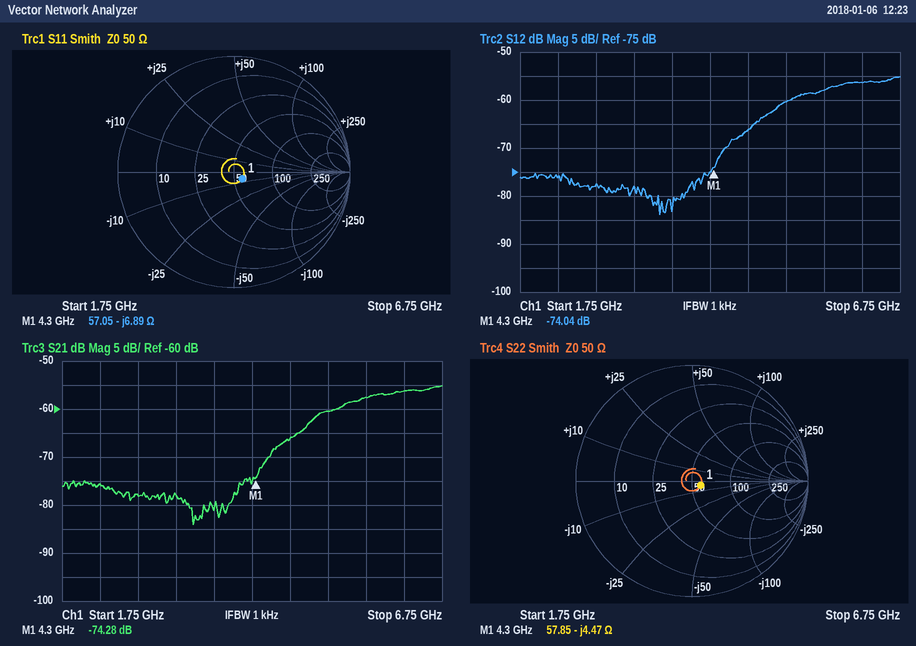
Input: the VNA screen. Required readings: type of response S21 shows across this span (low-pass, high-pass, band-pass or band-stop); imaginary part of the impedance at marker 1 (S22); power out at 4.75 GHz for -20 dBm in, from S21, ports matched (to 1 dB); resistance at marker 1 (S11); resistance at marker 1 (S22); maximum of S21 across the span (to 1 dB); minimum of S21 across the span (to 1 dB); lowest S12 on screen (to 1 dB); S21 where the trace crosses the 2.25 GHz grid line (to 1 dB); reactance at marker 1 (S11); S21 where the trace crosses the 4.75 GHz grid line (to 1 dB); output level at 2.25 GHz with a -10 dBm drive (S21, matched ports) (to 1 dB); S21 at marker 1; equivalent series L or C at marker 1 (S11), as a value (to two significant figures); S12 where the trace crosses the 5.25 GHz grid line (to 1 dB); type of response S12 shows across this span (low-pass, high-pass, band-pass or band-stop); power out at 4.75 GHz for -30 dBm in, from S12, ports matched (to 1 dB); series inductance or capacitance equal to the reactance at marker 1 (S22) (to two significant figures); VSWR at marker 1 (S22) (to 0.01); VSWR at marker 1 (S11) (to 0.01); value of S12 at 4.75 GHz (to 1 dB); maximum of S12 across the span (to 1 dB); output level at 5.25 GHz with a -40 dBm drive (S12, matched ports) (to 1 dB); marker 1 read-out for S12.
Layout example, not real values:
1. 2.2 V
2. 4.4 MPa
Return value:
1. high-pass
2. -4.47 Ω
3. -86 dBm
4. 57.05 Ω
5. 57.85 Ω
6. -55 dB
7. -84 dB
8. -84 dB
9. -76 dB
10. -6.89 Ω
11. -66 dB
12. -86 dBm
13. -74.28 dB
14. 5.4 pF
15. -60 dB
16. high-pass
17. -96 dBm
18. 8.3 pF
19. 1.18
20. 1.20
21. -66 dB
22. -55 dB
23. -100 dBm
24. -74.04 dB
